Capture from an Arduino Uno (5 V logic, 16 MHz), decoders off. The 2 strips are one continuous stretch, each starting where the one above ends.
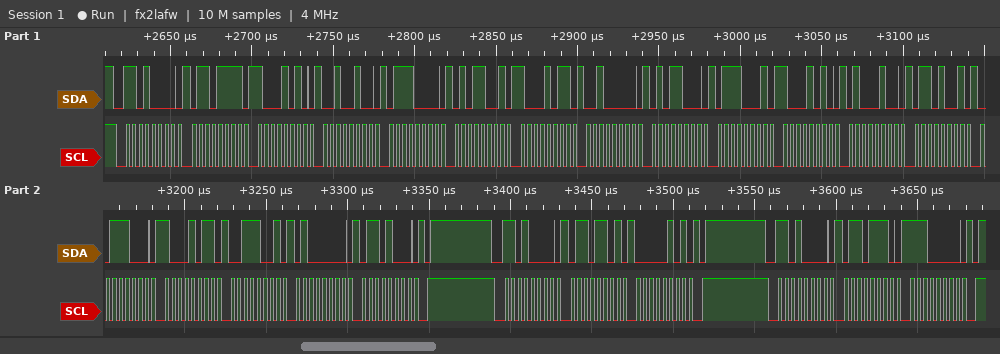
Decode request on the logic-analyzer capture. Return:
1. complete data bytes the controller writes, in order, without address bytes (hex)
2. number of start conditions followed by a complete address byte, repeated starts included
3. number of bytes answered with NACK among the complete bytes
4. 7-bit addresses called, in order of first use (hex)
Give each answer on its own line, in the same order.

6F 8A 24 70 59 8B 20 58 71 8A 44 69 38 8B 39 40 68 6D 05 6E E0
3
0
0x68
